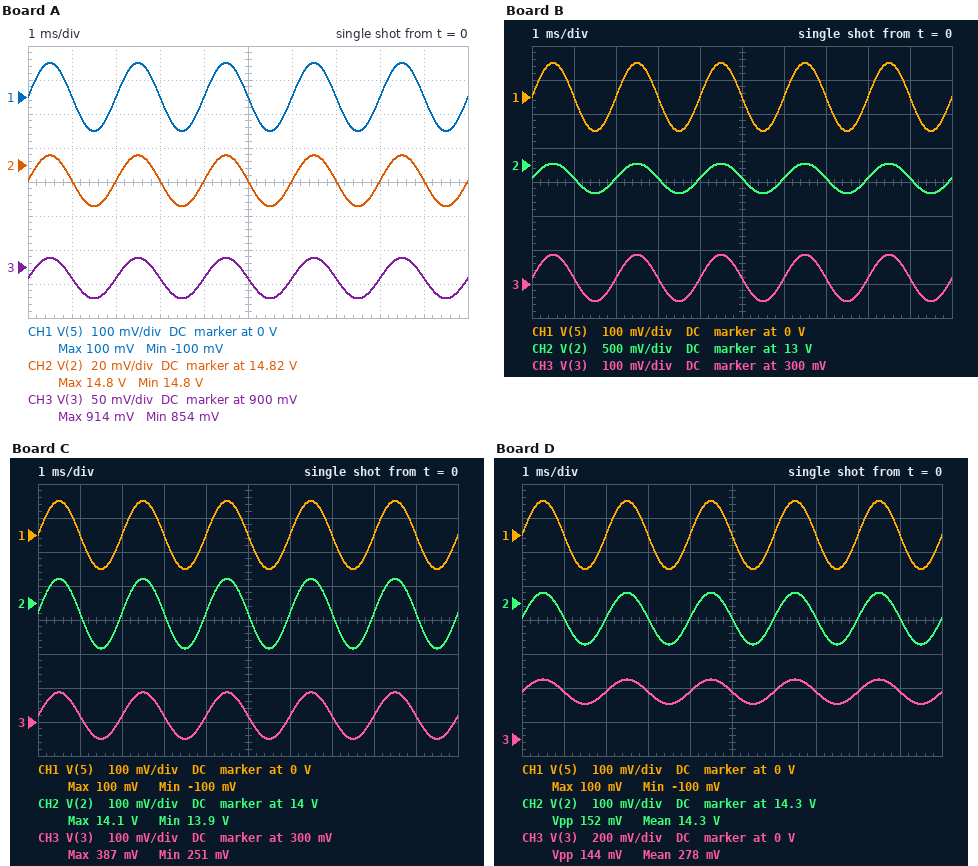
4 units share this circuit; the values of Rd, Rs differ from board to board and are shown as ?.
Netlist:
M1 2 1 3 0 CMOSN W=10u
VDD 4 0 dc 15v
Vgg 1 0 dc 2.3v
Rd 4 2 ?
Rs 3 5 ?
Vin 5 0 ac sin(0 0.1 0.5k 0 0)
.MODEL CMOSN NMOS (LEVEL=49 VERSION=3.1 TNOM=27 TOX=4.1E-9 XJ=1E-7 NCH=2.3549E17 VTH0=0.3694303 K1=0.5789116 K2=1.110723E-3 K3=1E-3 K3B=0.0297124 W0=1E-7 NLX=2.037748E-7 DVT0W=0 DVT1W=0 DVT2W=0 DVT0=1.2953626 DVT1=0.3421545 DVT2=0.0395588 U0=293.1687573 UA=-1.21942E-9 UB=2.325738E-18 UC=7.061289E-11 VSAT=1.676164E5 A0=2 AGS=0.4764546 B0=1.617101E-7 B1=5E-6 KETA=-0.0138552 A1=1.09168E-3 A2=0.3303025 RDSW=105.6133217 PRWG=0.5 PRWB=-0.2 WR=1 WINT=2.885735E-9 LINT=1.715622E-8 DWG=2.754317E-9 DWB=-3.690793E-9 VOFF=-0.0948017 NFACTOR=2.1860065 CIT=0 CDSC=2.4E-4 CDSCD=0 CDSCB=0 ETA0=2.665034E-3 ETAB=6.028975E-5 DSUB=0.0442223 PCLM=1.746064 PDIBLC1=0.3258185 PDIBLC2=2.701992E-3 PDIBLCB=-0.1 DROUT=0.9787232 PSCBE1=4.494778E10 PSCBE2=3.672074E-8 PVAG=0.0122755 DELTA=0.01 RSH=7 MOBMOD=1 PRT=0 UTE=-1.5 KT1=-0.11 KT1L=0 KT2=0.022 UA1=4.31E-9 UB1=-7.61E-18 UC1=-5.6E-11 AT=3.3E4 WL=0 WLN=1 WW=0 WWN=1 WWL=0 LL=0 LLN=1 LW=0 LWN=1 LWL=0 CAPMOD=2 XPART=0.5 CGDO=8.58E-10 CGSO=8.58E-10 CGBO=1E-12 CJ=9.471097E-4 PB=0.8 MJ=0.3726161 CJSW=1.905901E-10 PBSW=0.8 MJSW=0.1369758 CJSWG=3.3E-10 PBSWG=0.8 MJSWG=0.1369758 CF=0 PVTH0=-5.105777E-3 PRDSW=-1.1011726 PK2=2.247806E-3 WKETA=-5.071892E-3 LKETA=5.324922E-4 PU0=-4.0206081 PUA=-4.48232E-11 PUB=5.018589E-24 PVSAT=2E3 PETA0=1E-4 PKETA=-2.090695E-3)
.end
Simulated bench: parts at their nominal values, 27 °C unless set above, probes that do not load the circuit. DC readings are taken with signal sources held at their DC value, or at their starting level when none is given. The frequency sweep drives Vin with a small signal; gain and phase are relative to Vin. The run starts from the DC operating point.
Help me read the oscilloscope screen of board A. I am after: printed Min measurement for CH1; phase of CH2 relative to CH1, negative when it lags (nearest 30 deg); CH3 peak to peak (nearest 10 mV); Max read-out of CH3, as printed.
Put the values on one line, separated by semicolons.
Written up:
-100 mV; 0 deg; 60 mV; 914 mV
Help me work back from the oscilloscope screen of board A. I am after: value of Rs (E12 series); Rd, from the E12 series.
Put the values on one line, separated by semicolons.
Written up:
5.6 kΩ; 1.2 kΩ
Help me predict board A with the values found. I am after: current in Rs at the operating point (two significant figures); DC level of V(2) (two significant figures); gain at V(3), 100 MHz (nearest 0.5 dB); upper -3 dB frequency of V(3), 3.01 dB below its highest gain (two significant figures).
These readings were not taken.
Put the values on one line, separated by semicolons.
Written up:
160 µA; 15 V; -10.5 dB; 520 MHz
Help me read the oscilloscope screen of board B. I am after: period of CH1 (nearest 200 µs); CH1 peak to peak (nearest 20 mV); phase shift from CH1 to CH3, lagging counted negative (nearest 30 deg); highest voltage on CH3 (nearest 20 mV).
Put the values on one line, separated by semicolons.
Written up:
2.0 ms; 200 mV; 0 deg; 380 mV
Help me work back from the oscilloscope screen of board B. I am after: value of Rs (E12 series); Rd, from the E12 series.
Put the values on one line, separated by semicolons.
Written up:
680 Ω; 4.7 kΩ
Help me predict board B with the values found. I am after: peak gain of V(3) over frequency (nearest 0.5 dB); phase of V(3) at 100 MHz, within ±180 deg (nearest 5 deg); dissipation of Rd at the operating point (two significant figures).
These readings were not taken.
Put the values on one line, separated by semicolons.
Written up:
-3.5 dB; -5 deg; 1.0 mW
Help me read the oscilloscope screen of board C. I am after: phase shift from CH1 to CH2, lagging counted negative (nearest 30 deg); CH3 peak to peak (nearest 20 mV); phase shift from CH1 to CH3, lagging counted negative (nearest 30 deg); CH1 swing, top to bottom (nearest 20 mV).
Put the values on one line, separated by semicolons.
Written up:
0 deg; 140 mV; 0 deg; 200 mV
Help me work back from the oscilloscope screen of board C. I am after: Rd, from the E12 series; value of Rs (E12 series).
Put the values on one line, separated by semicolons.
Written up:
2.2 kΩ; 680 Ω
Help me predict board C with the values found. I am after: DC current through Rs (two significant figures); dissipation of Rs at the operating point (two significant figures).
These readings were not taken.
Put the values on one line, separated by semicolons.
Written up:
470 µA; 150 µW
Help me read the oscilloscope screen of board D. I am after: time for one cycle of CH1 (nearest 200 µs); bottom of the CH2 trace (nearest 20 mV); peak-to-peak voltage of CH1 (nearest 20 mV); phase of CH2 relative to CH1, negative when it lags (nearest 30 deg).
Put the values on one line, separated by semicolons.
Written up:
2.0 ms; 14.18 V; 200 mV; 0 deg
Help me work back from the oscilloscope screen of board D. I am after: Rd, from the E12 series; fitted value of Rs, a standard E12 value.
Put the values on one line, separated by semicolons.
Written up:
1.5 kΩ; 560 Ω
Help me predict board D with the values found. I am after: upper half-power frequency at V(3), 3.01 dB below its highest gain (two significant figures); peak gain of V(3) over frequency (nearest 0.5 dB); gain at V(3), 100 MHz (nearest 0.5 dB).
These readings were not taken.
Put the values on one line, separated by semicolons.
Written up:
2.1 GHz; -3.0 dB; -3.0 dB
